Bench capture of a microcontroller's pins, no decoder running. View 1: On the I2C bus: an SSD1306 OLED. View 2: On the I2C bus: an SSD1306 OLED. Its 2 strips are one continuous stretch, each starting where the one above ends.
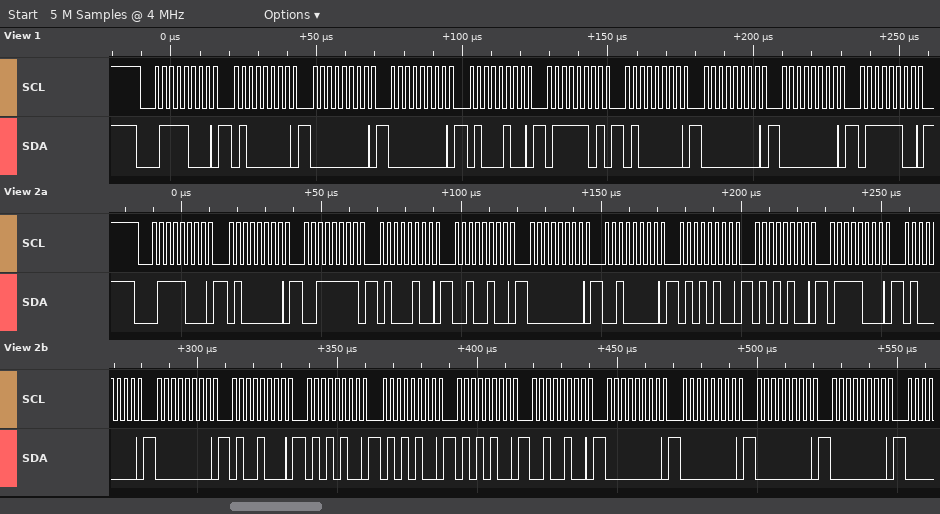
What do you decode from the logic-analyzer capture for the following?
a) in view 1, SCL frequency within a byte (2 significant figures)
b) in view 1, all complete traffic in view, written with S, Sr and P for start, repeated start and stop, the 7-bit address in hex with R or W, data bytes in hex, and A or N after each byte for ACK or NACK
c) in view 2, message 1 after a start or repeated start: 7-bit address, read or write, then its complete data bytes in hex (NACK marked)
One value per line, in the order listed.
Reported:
400 kHz
S 3CW A 40 A 00 A 00 A 44 A 7D A 40 A 00 A 00 A 7C A
0x3C write: 40 3F 44 24 00 20 54 54 78 40 00 48 54 54 54 24 00 00 00 00
